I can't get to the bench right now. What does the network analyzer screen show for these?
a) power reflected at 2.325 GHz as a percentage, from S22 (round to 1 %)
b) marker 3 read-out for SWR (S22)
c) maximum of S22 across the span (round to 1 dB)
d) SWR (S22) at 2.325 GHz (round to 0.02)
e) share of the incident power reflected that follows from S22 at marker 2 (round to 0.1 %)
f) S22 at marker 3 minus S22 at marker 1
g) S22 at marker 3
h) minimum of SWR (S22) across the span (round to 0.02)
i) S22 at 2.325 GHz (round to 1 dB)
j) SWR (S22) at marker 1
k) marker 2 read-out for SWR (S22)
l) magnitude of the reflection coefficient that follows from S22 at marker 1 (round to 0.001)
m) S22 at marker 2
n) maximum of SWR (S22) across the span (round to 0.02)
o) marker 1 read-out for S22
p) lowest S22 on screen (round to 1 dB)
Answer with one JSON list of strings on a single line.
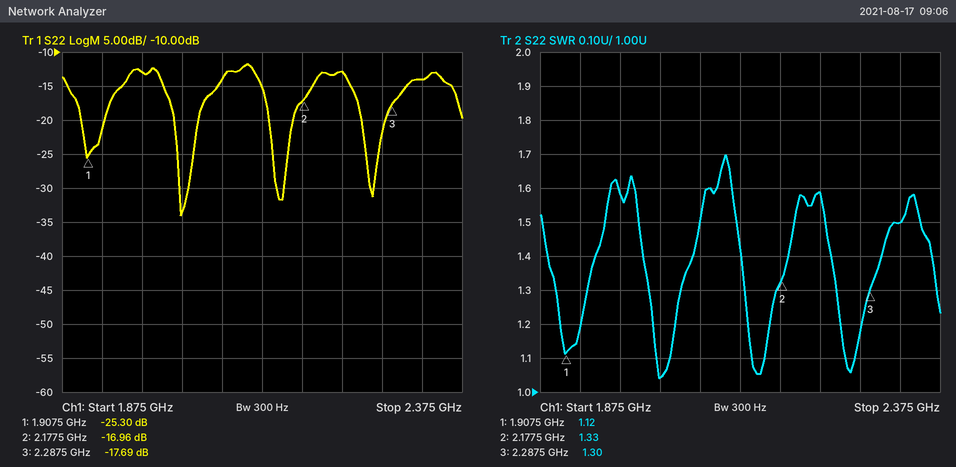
["4 %", "1.30", "-12 dB", "1.50", "2.0 %", "7.61 dB", "-17.69 dB", "1.04", "-14 dB", "1.12", "1.33", "0.054", "-16.96 dB", "1.70", "-25.30 dB", "-34 dB"]
